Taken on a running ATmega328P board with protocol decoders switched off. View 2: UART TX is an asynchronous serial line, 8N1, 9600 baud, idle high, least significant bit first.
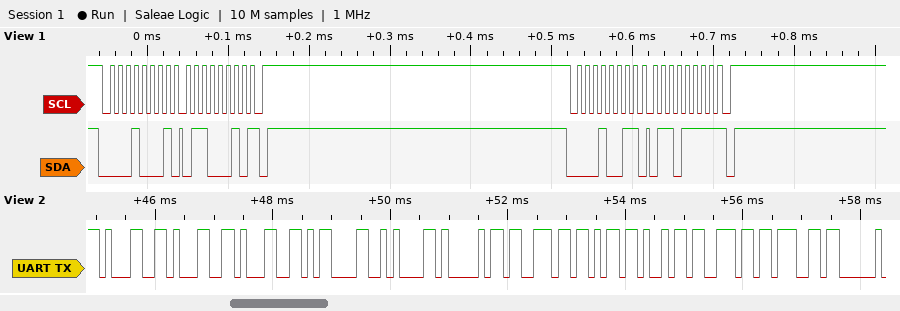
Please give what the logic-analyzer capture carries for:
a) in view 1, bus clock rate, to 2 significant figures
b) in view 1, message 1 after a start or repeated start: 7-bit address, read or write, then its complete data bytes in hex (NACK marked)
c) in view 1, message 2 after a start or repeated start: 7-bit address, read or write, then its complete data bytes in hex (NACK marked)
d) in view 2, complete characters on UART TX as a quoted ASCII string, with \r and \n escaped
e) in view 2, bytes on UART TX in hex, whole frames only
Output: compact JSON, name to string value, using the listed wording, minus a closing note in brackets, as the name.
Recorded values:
{"in view 1, bus clock rate, to 2 significant figures": "100 kHz", "in view 1, message 1 after a start or repeated start: 7-bit address, read or write, then its complete data bytes in hex": "0x08 read: 62 NACK", "in view 1, message 2 after a start or repeated start: 7-bit address, read or write, then its complete data bytes in hex": "0x09 read: 6F NACK", "in view 2, complete characters on UART TX as a quoted ASCII string, with \\r and \\n escaped": "\"111\\r\\nAsking\"", "in view 2, bytes on UART TX in hex, whole frames only": "31 31 31 0D 0A 41 73 6B 69 6E 67"}
